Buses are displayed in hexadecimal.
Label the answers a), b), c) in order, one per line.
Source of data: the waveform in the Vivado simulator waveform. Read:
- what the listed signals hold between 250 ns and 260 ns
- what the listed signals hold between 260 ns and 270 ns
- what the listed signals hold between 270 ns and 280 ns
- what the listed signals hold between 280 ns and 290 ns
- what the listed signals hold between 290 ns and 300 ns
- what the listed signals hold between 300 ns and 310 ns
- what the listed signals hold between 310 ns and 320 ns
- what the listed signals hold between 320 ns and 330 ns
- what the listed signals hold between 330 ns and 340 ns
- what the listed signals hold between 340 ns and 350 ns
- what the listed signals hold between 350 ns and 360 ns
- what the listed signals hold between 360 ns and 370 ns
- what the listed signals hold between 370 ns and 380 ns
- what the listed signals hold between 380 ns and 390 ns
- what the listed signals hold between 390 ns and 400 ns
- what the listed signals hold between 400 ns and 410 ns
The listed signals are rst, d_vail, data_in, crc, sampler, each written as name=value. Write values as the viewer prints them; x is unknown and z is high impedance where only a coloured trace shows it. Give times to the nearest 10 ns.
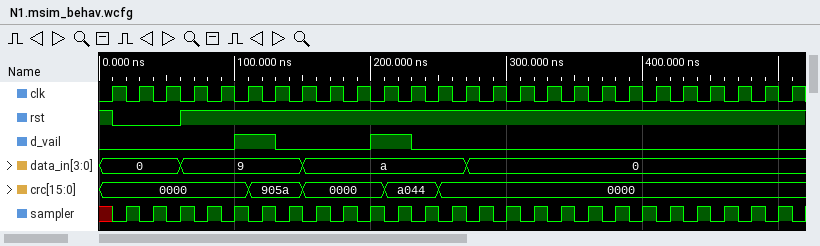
a) rst=1, d_vail=0, data_in=a, crc=0000, sampler=0
b) rst=1, d_vail=0, data_in=a, crc=0000, sampler=1
c) rst=1, d_vail=0, data_in=0, crc=0000, sampler=0
d) rst=1, d_vail=0, data_in=0, crc=0000, sampler=1
e) rst=1, d_vail=0, data_in=0, crc=0000, sampler=0
f) rst=1, d_vail=0, data_in=0, crc=0000, sampler=1
g) rst=1, d_vail=0, data_in=0, crc=0000, sampler=0
h) rst=1, d_vail=0, data_in=0, crc=0000, sampler=1
i) rst=1, d_vail=0, data_in=0, crc=0000, sampler=0
j) rst=1, d_vail=0, data_in=0, crc=0000, sampler=1
k) rst=1, d_vail=0, data_in=0, crc=0000, sampler=0
l) rst=1, d_vail=0, data_in=0, crc=0000, sampler=1
m) rst=1, d_vail=0, data_in=0, crc=0000, sampler=0
n) rst=1, d_vail=0, data_in=0, crc=0000, sampler=1
o) rst=1, d_vail=0, data_in=0, crc=0000, sampler=0
p) rst=1, d_vail=0, data_in=0, crc=0000, sampler=1
